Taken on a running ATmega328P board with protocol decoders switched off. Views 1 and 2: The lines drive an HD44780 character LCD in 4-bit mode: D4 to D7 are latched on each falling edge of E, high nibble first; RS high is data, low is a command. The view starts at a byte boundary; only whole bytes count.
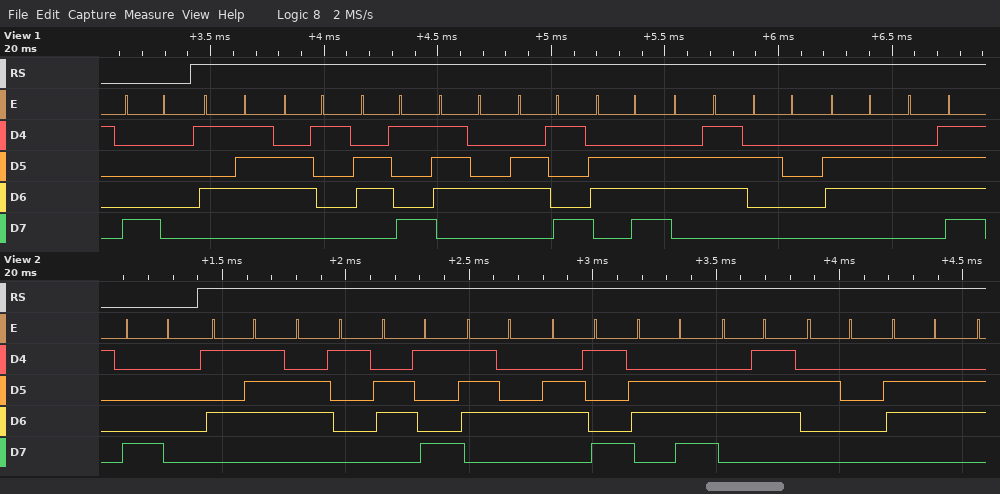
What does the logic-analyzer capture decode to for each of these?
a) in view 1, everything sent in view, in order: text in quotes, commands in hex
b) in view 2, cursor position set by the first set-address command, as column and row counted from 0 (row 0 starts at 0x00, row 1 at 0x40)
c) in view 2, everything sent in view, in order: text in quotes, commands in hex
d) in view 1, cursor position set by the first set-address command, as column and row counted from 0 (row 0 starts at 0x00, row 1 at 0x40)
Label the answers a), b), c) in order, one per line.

a) 0x80 "Waiting fo"
b) column 0, row 0
c) 0x80 "Waiting f"
d) column 0, row 0
